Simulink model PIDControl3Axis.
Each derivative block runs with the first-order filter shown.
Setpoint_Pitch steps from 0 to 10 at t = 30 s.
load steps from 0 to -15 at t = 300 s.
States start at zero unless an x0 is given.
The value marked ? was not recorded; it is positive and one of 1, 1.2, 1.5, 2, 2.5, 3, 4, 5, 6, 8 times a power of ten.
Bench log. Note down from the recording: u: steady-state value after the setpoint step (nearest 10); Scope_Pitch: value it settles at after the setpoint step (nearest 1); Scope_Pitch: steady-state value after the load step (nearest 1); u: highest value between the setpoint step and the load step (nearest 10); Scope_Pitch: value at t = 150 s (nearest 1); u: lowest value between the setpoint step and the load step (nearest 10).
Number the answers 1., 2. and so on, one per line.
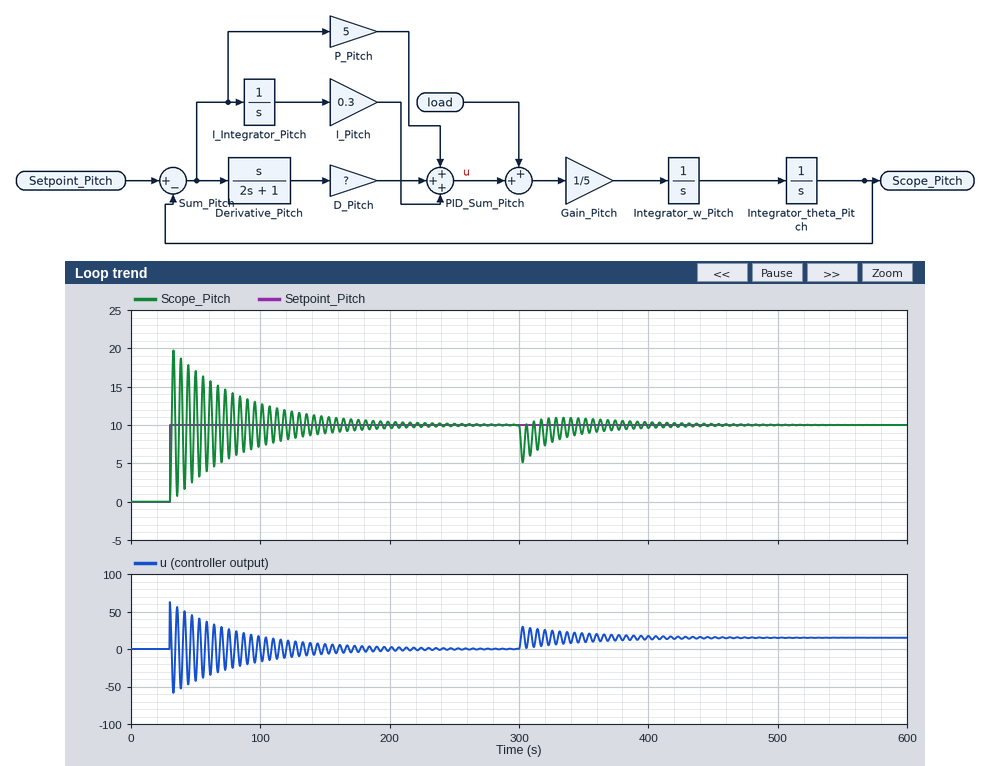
1. 0
2. 10
3. 10
4. 60
5. 9
6. -60
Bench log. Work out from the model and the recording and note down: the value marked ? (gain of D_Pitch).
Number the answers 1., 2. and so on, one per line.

1. 2.5
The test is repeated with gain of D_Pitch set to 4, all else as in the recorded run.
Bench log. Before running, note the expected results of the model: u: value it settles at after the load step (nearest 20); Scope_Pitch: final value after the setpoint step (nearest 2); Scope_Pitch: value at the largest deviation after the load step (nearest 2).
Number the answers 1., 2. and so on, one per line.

1. 20
2. 10
3. 6
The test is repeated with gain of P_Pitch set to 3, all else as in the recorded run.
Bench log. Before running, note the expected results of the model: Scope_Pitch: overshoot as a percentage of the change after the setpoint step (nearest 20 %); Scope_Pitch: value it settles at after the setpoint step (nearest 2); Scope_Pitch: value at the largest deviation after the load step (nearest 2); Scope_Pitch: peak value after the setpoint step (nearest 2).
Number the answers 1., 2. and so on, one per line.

1. 100 %
2. 10
3. 2
4. 20
